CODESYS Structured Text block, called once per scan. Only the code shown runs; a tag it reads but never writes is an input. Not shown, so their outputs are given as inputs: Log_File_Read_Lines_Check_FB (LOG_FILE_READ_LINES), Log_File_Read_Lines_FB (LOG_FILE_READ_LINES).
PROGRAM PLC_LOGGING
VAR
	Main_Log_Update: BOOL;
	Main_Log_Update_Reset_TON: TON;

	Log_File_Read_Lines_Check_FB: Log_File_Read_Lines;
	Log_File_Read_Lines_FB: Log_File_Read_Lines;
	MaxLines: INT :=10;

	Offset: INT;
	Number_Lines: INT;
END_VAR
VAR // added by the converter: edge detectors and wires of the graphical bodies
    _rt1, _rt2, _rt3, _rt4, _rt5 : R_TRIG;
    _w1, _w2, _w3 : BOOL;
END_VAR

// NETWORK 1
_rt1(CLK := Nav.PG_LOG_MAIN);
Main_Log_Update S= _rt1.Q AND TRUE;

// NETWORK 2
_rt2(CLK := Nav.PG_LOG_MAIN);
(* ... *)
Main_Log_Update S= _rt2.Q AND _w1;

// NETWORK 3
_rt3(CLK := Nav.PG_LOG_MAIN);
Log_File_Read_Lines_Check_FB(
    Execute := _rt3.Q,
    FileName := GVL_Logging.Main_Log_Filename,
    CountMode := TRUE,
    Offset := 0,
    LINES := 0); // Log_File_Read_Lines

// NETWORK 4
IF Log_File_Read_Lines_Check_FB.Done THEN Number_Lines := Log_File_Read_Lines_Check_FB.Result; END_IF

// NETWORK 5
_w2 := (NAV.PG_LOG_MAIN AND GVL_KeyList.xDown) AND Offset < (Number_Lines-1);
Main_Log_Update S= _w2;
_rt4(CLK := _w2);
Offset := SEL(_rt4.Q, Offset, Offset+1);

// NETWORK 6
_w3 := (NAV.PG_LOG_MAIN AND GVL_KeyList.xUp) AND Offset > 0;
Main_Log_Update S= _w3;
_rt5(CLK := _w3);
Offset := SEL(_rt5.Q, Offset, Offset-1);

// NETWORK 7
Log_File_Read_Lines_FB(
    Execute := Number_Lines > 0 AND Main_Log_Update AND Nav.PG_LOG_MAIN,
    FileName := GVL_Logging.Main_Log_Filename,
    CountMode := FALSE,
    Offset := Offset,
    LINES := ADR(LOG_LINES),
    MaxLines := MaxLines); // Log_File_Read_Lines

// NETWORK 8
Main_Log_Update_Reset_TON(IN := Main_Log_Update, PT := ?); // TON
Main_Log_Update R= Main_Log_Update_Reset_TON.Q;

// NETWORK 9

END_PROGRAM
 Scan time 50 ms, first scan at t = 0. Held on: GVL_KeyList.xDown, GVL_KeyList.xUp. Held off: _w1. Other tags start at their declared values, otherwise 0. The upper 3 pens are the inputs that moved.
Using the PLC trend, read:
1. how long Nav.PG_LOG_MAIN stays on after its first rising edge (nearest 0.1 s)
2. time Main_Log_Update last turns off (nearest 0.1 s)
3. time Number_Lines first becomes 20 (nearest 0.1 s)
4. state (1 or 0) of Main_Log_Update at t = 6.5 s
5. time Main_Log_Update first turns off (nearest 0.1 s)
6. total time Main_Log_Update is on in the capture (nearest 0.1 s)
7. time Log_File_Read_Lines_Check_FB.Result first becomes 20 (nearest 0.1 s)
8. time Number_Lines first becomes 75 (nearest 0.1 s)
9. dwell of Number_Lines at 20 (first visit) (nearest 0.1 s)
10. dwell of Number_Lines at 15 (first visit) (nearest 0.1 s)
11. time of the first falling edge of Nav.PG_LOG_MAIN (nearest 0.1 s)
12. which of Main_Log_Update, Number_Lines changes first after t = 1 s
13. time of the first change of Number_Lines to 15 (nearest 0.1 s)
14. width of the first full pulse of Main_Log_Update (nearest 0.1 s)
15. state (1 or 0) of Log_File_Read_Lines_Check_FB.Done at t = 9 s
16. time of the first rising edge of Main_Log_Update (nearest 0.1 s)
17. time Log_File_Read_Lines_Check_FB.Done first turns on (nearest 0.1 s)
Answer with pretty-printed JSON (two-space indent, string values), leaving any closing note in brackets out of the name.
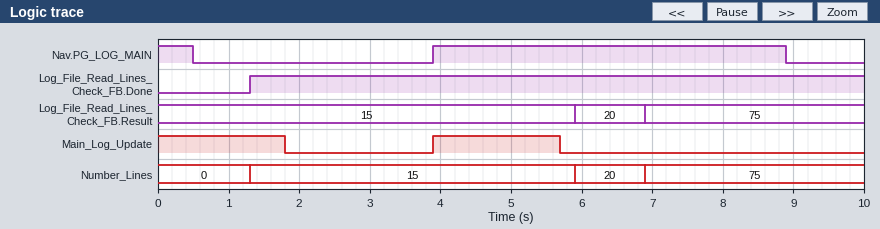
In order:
{
  "how long Nav.PG_LOG_MAIN stays on after its first rising edge": "5.0 s",
  "time Main_Log_Update last turns off": "5.7 s",
  "time Number_Lines first becomes 20": "5.9 s",
  "state (1 or 0) of Main_Log_Update at t = 6.5 s": "0",
  "time Main_Log_Update first turns off": "1.8 s",
  "total time Main_Log_Update is on in the capture": "3.6 s",
  "time Log_File_Read_Lines_Check_FB.Result first becomes 20": "5.9 s",
  "time Number_Lines first becomes 75": "6.9 s",
  "dwell of Number_Lines at 20 (first visit)": "1.0 s",
  "dwell of Number_Lines at 15 (first visit)": "4.6 s",
  "time of the first falling edge of Nav.PG_LOG_MAIN": "0.5 s",
  "which of Main_Log_Update, Number_Lines changes first after t = 1 s": "Number_Lines",
  "time of the first change of Number_Lines to 15": "1.3 s",
  "width of the first full pulse of Main_Log_Update": "1.8 s",
  "state (1 or 0) of Log_File_Read_Lines_Check_FB.Done at t = 9 s": "1",
  "time of the first rising edge of Main_Log_Update": "3.9 s",
  "time Log_File_Read_Lines_Check_FB.Done first turns on": "1.3 s"
}
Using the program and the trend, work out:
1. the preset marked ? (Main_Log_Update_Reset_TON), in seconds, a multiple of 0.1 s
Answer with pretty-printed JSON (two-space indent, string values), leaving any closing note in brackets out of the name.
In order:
{
  "the preset marked ? (Main_Log_Update_Reset_TON), in seconds, a multiple of 0.1 s": "1.8 s"
}
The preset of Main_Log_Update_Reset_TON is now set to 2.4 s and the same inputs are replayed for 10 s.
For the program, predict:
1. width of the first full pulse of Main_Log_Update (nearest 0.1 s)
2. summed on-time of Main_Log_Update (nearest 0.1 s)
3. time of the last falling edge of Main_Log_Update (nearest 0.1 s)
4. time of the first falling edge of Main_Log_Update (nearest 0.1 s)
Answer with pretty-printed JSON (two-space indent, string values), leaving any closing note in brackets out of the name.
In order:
{
  "width of the first full pulse of Main_Log_Update": "2.4 s",
  "summed on-time of Main_Log_Update": "4.8 s",
  "time of the last falling edge of Main_Log_Update": "6.3 s",
  "time of the first falling edge of Main_Log_Update": "2.4 s"
}
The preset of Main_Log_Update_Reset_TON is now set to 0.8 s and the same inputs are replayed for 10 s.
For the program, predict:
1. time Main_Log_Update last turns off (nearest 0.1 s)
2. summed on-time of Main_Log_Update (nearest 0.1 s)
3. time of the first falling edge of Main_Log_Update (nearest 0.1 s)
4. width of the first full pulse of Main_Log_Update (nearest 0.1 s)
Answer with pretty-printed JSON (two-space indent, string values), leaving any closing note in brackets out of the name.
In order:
{
  "time Main_Log_Update last turns off": "4.7 s",
  "summed on-time of Main_Log_Update": "1.6 s",
  "time of the first falling edge of Main_Log_Update": "0.8 s",
  "width of the first full pulse of Main_Log_Update": "0.8 s"
}
